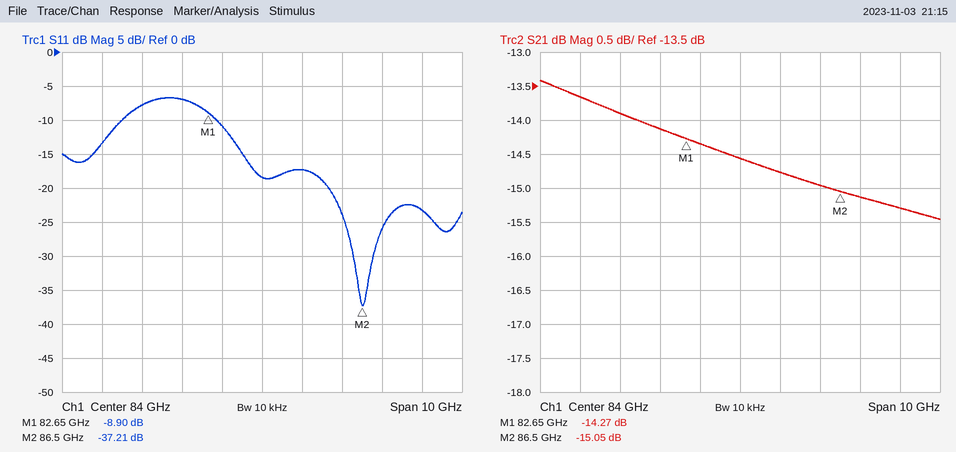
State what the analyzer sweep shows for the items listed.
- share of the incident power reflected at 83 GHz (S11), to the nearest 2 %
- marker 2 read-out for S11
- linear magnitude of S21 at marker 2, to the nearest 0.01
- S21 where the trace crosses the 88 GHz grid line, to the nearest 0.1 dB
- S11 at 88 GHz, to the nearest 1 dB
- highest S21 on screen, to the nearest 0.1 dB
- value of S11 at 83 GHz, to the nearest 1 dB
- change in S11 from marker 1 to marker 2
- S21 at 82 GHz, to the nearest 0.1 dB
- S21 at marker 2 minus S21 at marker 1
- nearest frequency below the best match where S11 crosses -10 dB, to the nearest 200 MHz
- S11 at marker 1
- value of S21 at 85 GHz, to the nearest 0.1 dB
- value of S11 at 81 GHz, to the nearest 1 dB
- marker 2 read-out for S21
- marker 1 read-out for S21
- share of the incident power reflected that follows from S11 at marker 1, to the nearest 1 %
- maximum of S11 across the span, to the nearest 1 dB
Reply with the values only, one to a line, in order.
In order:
8 %
-37.21 dB
0.18
-15.3 dB
-23 dB
-13.4 dB
-11 dB
-28.31 dB
-14.1 dB
-0.78 dB
82.8 GHz
-8.90 dB
-14.8 dB
-8 dB
-15.05 dB
-14.27 dB
13 %
-7 dB
